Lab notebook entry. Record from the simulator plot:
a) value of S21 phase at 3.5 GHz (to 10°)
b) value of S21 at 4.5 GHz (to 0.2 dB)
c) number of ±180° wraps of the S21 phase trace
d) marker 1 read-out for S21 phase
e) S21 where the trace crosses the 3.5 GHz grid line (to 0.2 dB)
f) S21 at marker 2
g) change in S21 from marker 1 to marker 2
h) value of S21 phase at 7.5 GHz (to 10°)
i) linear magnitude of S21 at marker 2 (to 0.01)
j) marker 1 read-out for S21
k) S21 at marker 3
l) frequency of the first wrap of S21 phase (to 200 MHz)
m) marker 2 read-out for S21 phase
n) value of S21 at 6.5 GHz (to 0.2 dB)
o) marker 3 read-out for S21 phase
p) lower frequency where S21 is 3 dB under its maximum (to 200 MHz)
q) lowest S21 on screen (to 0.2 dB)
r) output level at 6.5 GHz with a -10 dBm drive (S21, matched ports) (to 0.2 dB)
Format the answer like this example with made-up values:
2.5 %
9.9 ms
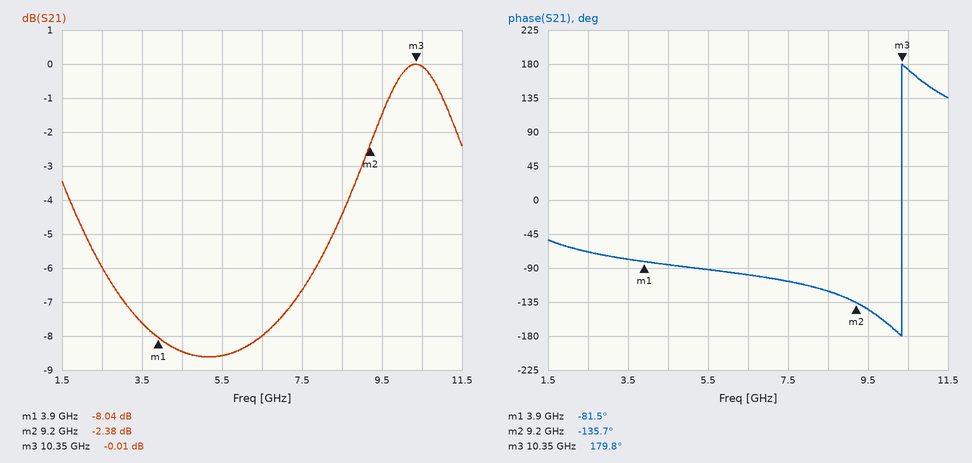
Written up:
-80°
-8.4 dB
1
-81.5°
-7.6 dB
-2.38 dB
5.66 dB
-110°
0.76
-8.04 dB
-0.01 dB
10.4 GHz
-135.7°
-8.0 dB
179.8°
9.0 GHz
-8.6 dB
-18.0 dBm
